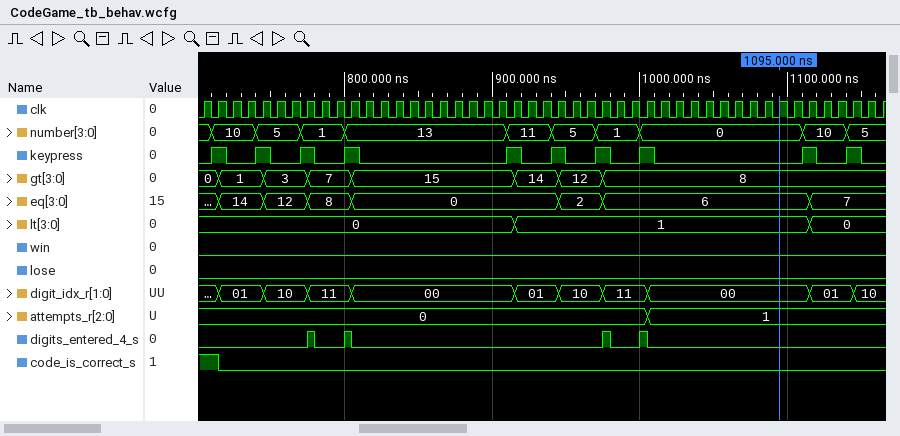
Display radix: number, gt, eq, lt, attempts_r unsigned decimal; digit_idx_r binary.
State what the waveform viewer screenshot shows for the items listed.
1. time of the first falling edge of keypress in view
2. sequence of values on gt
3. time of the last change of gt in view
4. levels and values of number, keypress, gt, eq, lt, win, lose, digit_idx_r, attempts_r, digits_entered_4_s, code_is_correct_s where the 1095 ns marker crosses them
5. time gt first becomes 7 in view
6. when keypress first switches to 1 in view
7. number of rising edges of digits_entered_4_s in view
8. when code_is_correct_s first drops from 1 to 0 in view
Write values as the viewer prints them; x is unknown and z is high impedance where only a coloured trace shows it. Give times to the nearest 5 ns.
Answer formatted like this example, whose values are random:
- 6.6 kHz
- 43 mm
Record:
- 720 ns
- 0, 1, 3, 7, 15, 14, 12, 8
- 975 ns
- number=0, keypress=0, gt=8, eq=6, lt=1, win=0, lose=0, digit_idx_r=00, attempts_r=1, digits_entered_4_s=0, code_is_correct_s=0
- 775 ns
- 710 ns
- 4
- 715 ns
